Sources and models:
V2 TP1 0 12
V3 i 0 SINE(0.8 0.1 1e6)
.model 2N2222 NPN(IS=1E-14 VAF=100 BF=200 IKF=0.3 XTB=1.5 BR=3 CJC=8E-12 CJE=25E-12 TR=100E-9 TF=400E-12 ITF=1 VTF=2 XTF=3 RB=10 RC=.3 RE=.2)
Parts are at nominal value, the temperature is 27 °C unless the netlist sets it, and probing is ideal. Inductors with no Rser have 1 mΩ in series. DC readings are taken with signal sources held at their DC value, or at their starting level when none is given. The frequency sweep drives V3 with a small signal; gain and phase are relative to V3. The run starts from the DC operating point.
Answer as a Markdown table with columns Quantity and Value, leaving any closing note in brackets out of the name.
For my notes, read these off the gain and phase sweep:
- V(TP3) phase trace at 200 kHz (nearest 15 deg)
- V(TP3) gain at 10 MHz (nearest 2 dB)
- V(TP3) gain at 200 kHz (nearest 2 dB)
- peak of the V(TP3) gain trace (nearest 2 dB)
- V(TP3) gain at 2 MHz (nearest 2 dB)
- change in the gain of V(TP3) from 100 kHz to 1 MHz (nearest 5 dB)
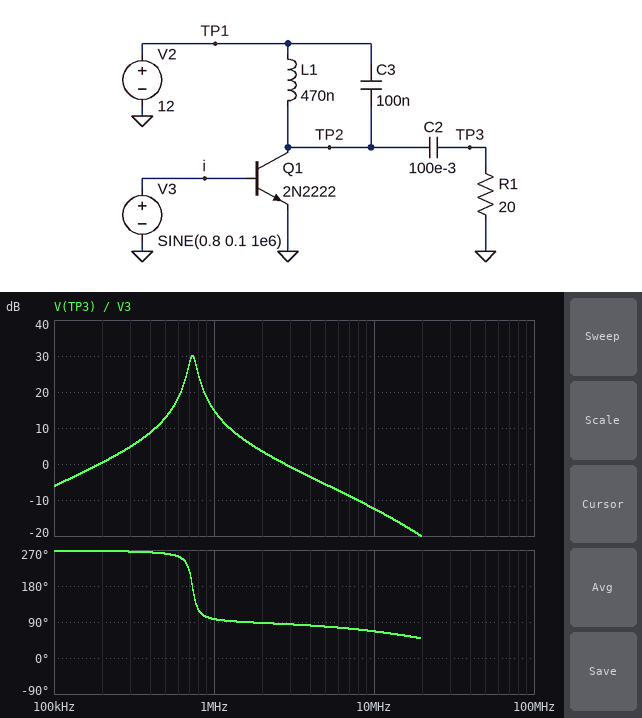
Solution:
| Quantity | Value |
|---|---|
| V(TP3) phase trace at 200 kHz | 270 deg |
| V(TP3) gain at 10 MHz | -12 dB |
| V(TP3) gain at 200 kHz | 0 dB |
| peak of the V(TP3) gain trace | 30 dB |
| V(TP3) gain at 2 MHz | 4 dB |
| change in the gain of V(TP3) from 100 kHz to 1 MHz | 20 dB |
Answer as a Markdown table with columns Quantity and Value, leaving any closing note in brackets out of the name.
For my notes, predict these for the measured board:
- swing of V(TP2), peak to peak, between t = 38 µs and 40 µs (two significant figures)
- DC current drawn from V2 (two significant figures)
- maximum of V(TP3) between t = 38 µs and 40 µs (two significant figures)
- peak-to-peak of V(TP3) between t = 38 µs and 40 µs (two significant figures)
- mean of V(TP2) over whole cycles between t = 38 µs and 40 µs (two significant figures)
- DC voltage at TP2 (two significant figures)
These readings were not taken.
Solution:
| Quantity | Value |
|---|---|
| swing of V(TP2), peak to peak, between t = 38 µs and 40 µs | 1.0 V |
| DC current drawn from V2 | 93 mA |
| maximum of V(TP3) between t = 38 µs and 40 µs | 500 mV |
| peak-to-peak of V(TP3) between t = 38 µs and 40 µs | 1.0 V |
| mean of V(TP2) over whole cycles between t = 38 µs and 40 µs | 12 V |
| DC voltage at TP2 | 12 V |
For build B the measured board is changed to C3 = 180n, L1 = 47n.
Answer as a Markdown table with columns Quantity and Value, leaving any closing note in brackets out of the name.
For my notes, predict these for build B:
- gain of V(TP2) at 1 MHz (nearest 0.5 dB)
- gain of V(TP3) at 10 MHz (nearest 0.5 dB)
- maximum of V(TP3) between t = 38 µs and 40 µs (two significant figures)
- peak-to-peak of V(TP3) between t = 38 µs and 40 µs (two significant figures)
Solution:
| Quantity | Value |
|---|---|
| gain of V(TP2) at 1 MHz | -3.0 dB |
| gain of V(TP3) at 10 MHz | -17.5 dB |
| maximum of V(TP3) between t = 38 µs and 40 µs | 100 mV |
| peak-to-peak of V(TP3) between t = 38 µs and 40 µs | 200 mV |
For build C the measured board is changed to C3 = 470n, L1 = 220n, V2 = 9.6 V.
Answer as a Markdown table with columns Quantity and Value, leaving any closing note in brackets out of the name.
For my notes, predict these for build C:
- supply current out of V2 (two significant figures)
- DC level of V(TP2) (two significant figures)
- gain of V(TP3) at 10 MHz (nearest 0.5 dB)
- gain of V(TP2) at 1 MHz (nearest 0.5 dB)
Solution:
| Quantity | Value |
|---|---|
| supply current out of V2 | 92 mA |
| DC level of V(TP2) | 9.6 V |
| gain of V(TP3) at 10 MHz | -26.0 dB |
| gain of V(TP2) at 1 MHz | -3.0 dB |
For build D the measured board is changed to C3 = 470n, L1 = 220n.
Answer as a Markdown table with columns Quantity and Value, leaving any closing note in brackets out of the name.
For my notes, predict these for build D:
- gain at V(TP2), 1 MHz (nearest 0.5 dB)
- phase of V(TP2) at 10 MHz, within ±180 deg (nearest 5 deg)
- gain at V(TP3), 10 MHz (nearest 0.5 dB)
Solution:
| Quantity | Value |
|---|---|
| gain at V(TP2), 1 MHz | -2.5 dB |
| phase of V(TP2) at 10 MHz, within ±180 deg | 65 deg |
| gain at V(TP3), 10 MHz | -26.0 dB |
